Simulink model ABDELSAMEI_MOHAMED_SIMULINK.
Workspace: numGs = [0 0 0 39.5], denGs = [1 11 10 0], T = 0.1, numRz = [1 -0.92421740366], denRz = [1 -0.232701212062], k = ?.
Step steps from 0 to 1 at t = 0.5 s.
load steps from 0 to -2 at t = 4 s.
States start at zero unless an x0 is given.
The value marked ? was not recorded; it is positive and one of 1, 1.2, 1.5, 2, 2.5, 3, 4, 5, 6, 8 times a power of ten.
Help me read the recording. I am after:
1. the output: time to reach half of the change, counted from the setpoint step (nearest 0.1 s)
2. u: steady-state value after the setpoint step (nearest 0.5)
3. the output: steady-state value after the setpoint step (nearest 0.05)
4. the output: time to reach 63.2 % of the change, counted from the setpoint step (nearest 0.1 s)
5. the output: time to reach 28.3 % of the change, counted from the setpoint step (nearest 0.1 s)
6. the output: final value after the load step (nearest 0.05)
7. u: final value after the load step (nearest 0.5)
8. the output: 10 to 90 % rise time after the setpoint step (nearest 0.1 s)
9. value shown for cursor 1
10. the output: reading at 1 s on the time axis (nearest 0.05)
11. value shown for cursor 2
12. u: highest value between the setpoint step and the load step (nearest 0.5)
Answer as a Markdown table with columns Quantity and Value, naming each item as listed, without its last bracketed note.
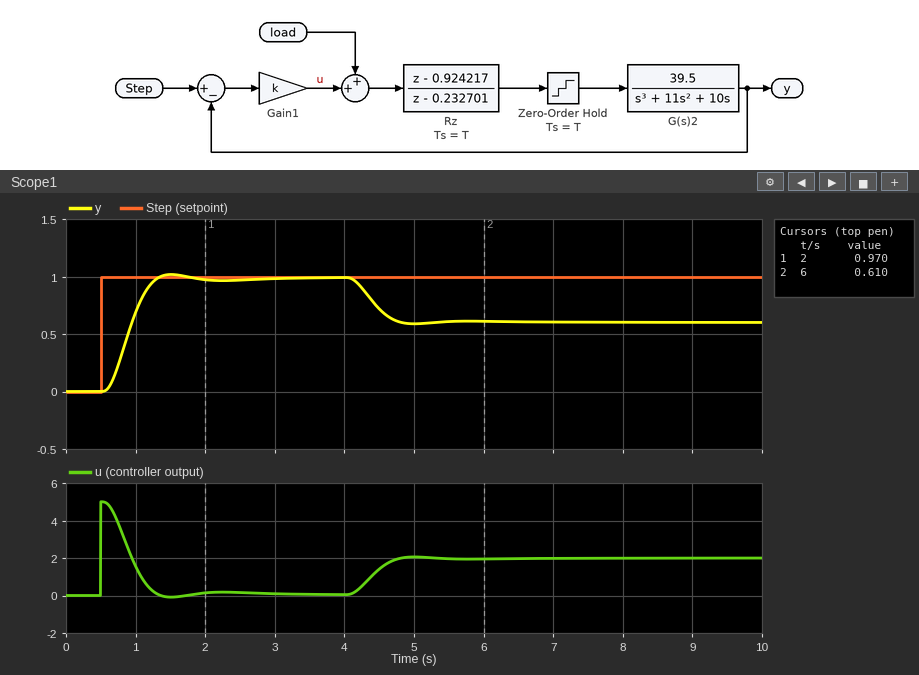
| Quantity | Value |
|---|---|
| the output: time to reach half of the change, counted from the setpoint step | 0.4 s |
| u: steady-state value after the setpoint step | 0.0 |
| the output: steady-state value after the setpoint step | 1.00 |
| the output: time to reach 63.2 % of the change, counted from the setpoint step | 0.5 s |
| the output: time to reach 28.3 % of the change, counted from the setpoint step | 0.3 s |
| the output: final value after the load step | 0.60 |
| u: final value after the load step | 2.0 |
| the output: 10 to 90 % rise time after the setpoint step | 0.5 s |
| value shown for cursor 1 | 0.970 |
| the output: reading at 1 s on the time axis | 0.70 |
| value shown for cursor 2 | 0.610 |
| u: highest value between the setpoint step and the load step | 5.0 |
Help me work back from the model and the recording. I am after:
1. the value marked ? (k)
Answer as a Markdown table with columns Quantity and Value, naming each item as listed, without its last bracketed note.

| Quantity | Value |
|---|---|
| the value marked ? | 5 |
